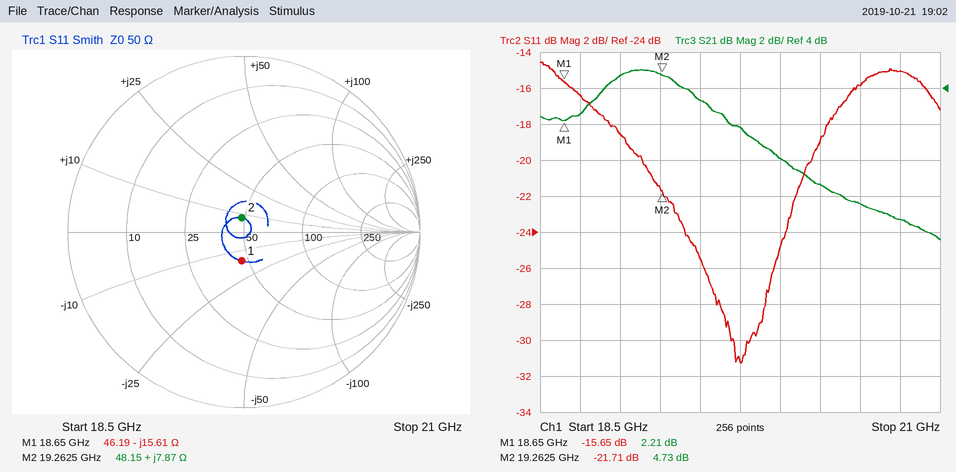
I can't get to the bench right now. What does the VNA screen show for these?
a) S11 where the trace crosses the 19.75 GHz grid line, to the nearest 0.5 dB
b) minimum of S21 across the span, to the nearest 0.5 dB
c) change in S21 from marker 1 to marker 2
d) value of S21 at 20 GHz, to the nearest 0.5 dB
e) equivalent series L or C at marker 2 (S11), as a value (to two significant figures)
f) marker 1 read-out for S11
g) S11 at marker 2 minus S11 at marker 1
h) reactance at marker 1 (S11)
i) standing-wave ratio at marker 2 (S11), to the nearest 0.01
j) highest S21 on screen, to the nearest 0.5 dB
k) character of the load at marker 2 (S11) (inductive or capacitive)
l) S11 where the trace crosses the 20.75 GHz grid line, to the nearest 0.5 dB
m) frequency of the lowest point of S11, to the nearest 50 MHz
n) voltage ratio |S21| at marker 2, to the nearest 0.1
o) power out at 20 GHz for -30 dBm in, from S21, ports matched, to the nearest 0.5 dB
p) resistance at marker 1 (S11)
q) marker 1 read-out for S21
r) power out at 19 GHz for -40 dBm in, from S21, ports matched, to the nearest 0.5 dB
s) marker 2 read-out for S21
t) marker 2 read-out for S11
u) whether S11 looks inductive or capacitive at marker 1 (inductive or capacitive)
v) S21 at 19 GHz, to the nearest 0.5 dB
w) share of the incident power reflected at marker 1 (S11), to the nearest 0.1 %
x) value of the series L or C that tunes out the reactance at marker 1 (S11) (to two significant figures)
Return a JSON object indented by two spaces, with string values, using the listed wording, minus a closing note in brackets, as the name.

{
  "S11 where the trace crosses the 19.75 GHz grid line, to the nearest 0.5 dB": "-31.0 dB",
  "minimum of S21 across the span, to the nearest 0.5 dB": "-4.5 dB",
  "change in S21 from marker 1 to marker 2": "2.52 dB",
  "value of S21 at 20 GHz, to the nearest 0.5 dB": "0.0 dB",
  "equivalent series L or C at marker 2 (S11), as a value": "65 pH",
  "marker 1 read-out for S11": "-15.65 dB",
  "S11 at marker 2 minus S11 at marker 1": "-6.06 dB",
  "reactance at marker 1": "-15.61 Ω",
  "standing-wave ratio at marker 2 (S11), to the nearest 0.01": "1.18",
  "highest S21 on screen, to the nearest 0.5 dB": "5.0 dB",
  "character of the load at marker 2 (S11)": "inductive",
  "S11 where the trace crosses the 20.75 GHz grid line, to the nearest 0.5 dB": "-15.0 dB",
  "frequency of the lowest point of S11, to the nearest 50 MHz": "19.75 GHz",
  "voltage ratio |S21| at marker 2, to the nearest 0.1": "1.7",
  "power out at 20 GHz for -30 dBm in, from S21, ports matched, to the nearest 0.5 dB": "-30.0 dBm",
  "resistance at marker 1": "46.19 Ω",
  "marker 1 read-out for S21": "2.21 dB",
  "power out at 19 GHz for -40 dBm in, from S21, ports matched, to the nearest 0.5 dB": "-35.5 dBm",
  "marker 2 read-out for S21": "4.73 dB",
  "marker 2 read-out for S11": "-21.71 dB",
  "whether S11 looks inductive or capacitive at marker 1": "capacitive",
  "S21 at 19 GHz, to the nearest 0.5 dB": "4.5 dB",
  "share of the incident power reflected at marker 1 (S11), to the nearest 0.1 %": "2.7 %",
  "value of the series L or C that tunes out the reactance at marker 1 (S11)": "130 pH"
}
